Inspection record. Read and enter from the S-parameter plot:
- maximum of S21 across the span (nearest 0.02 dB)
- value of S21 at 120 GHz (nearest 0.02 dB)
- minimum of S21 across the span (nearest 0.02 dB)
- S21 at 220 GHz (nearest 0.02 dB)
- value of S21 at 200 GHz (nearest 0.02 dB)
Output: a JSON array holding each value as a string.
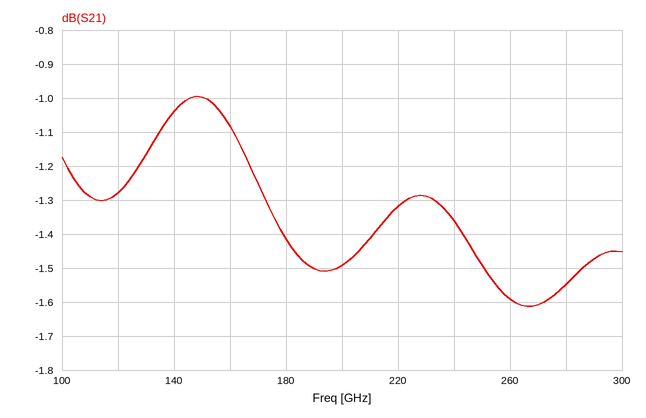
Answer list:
["-1.00 dB", "-1.28 dB", "-1.62 dB", "-1.32 dB", "-1.50 dB"]
